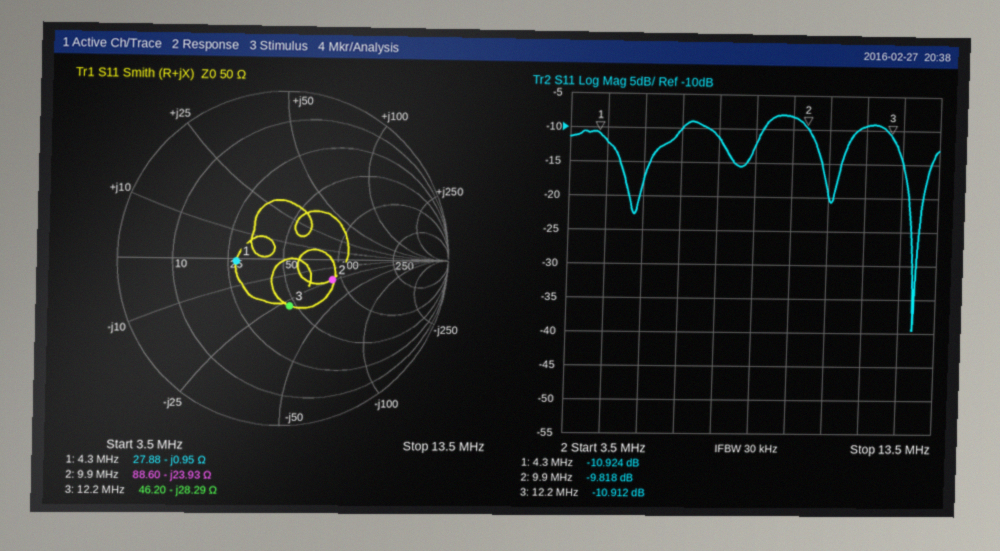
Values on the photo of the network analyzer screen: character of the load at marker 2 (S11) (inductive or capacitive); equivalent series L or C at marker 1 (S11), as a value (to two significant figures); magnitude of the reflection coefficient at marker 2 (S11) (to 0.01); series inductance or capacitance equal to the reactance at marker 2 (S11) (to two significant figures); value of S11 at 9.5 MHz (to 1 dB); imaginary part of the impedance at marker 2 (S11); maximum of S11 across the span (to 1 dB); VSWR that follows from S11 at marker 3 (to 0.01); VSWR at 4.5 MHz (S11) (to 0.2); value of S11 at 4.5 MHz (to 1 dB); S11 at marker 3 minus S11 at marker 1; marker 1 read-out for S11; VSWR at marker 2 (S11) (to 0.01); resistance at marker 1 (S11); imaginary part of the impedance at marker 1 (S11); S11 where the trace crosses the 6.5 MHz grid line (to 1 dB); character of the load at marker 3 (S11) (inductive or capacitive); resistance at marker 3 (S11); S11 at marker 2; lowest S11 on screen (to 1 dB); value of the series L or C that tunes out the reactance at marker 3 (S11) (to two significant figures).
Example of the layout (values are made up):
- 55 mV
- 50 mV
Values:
- capacitive
- 39 nF
- 0.32
- 670 pF
- -8 dB
- -23.93 Ω
- -8 dB
- 1.80
- 1.6
- -12 dB
- 0.012 dB
- -10.924 dB
- 1.95
- 27.88 Ω
- -0.95 Ω
- -10 dB
- capacitive
- 46.20 Ω
- -9.818 dB
- -40 dB
- 370 nH
